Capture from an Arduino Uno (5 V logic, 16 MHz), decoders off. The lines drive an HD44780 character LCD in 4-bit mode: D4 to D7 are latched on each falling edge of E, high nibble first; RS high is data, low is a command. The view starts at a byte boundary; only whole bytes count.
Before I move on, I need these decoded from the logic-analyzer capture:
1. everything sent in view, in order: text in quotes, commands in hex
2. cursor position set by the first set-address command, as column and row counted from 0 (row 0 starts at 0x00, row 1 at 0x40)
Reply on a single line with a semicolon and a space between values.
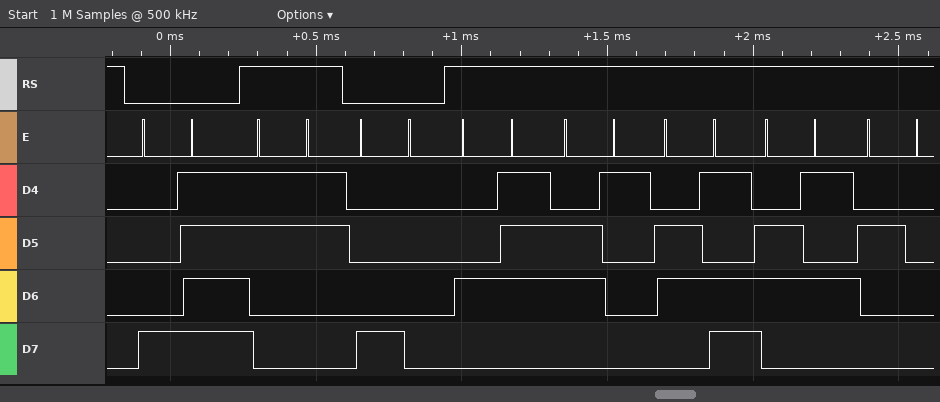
0x8F "3" 0x80 "Game "; column 15, row 0
